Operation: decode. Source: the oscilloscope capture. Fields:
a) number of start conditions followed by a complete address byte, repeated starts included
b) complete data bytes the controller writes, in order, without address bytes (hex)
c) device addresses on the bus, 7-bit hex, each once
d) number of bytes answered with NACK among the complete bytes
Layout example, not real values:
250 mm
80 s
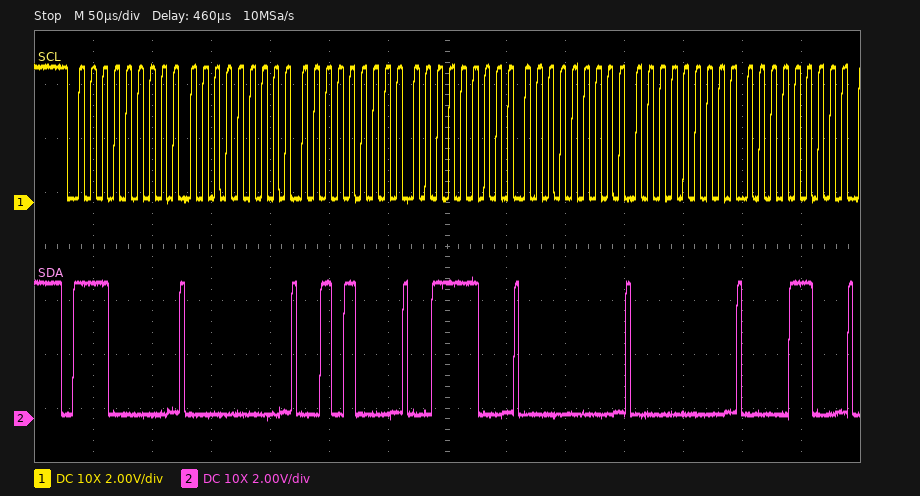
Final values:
1
00 28 3C 00 00 0C
0x70
0
